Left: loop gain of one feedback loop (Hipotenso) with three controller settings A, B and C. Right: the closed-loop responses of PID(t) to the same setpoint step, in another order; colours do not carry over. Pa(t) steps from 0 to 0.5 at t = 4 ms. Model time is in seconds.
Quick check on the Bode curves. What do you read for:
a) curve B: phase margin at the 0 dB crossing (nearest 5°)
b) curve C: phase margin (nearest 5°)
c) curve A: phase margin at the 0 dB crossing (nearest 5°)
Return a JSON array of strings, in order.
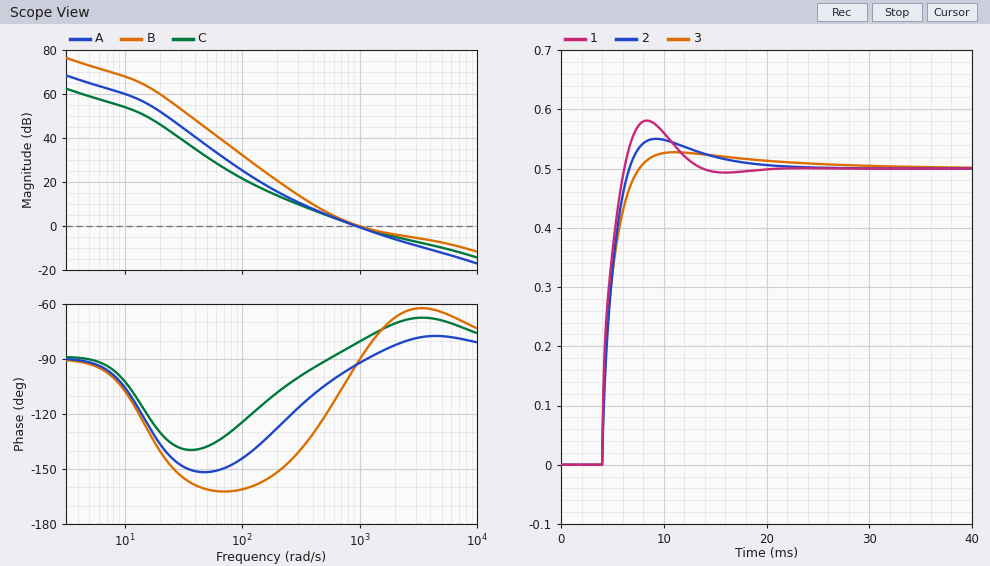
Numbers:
["90°", "100°", "85°"]
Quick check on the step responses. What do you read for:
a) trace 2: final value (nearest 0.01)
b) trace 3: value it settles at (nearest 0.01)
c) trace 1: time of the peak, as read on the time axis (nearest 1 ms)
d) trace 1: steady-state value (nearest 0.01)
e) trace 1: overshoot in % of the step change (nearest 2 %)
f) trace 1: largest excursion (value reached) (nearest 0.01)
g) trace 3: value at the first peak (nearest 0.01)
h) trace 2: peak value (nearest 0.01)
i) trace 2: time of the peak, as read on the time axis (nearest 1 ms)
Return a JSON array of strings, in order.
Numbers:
["0.50", "0.50", "8 ms", "0.50", "16 %", "0.58", "0.53", "0.55", "9 ms"]
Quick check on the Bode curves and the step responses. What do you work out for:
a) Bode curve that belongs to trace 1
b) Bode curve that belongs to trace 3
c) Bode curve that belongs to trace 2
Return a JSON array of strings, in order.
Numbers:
["B", "C", "A"]
